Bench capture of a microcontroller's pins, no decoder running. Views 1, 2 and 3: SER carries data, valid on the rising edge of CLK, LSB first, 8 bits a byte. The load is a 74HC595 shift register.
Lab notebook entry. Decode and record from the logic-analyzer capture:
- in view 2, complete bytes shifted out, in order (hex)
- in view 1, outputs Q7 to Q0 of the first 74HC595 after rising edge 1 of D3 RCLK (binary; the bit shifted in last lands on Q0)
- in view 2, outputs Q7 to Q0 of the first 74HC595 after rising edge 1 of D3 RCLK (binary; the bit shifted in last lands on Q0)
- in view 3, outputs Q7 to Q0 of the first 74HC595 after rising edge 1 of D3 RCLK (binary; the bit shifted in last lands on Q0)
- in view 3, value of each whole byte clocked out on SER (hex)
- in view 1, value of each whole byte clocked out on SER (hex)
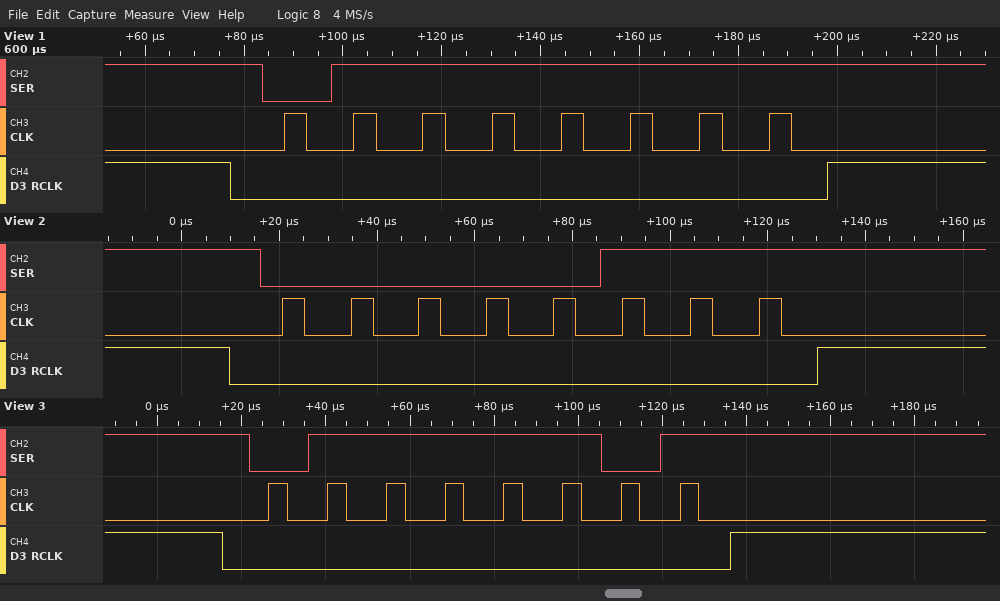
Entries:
E0
01111111
00000111
01111101
0xBE
FE
